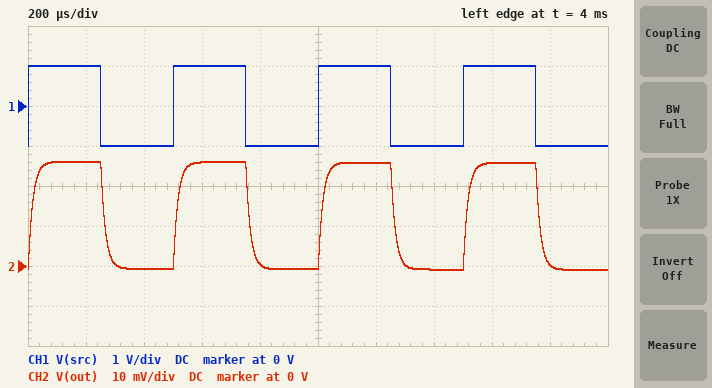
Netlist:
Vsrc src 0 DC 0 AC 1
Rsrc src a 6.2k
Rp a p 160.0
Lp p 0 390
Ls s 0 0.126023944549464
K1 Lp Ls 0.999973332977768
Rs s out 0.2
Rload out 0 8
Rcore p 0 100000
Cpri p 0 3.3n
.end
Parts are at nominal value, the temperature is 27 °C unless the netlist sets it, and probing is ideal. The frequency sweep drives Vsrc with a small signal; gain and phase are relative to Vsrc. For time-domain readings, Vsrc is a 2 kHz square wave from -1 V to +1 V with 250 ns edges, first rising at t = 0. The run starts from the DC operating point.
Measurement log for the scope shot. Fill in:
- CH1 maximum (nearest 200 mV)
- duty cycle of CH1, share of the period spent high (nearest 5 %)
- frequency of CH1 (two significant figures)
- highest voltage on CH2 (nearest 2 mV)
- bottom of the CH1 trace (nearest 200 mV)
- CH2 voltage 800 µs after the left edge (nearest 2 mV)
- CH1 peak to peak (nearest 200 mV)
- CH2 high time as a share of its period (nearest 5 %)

1.0 V
50 %
2.0 kHz
26 mV
-1.0 V
0 V
2.0 V
50 %
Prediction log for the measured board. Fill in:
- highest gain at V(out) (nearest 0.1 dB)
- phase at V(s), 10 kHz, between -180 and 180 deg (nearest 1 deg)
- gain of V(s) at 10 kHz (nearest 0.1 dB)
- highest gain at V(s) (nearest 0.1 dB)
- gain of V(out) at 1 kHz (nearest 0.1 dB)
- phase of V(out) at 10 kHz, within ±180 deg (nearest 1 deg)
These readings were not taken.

-37.5 dB
-48 deg
-40.3 dB
-37.3 dB
-37.5 dB
-48 deg
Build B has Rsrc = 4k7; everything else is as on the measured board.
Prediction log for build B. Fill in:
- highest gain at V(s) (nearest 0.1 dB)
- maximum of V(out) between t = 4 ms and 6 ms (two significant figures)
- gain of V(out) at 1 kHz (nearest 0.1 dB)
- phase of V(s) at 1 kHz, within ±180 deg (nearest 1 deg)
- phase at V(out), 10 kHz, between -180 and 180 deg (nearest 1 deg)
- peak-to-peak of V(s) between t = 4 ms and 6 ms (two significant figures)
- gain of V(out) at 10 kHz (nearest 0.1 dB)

-36.8 dB
28 mV
-37.0 dB
-5 deg
-42 deg
29 mV
-39.2 dB
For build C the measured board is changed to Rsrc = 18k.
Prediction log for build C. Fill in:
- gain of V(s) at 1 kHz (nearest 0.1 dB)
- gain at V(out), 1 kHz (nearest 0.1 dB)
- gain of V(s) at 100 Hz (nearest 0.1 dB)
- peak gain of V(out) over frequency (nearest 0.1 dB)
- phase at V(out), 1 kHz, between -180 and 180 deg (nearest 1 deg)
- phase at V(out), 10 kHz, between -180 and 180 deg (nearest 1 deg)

-40.6 dB
-40.8 dB
-40.5 dB
-40.7 dB
-11 deg
-66 deg
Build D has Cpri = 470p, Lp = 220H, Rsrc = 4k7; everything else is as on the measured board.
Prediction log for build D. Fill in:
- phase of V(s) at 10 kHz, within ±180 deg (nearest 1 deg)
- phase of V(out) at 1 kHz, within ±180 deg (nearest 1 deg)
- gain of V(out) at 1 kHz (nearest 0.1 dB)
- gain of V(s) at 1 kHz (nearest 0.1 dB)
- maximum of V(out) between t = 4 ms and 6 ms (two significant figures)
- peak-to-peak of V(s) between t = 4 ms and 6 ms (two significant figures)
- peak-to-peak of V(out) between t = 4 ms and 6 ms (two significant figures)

-8 deg
-1 deg
-35.5 dB
-35.3 dB
33 mV
35 mV
34 mV
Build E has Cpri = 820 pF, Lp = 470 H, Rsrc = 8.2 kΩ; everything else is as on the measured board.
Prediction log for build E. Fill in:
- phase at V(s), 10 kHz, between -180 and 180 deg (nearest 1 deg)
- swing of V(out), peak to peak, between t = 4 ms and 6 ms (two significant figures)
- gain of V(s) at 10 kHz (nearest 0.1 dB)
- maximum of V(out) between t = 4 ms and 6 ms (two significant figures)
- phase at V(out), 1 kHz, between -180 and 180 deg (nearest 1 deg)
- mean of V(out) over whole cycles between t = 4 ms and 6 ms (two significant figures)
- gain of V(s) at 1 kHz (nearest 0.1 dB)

-20 deg
24 mV
-38.8 dB
23 mV
-2 deg
11 mV
-38.4 dB
